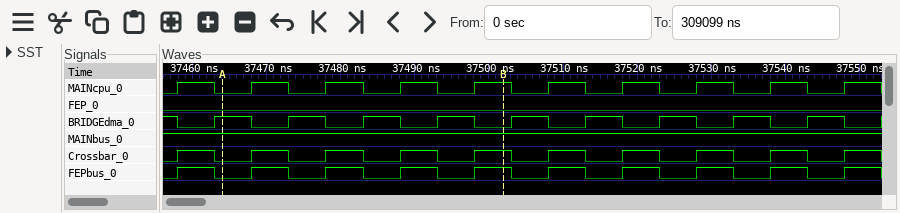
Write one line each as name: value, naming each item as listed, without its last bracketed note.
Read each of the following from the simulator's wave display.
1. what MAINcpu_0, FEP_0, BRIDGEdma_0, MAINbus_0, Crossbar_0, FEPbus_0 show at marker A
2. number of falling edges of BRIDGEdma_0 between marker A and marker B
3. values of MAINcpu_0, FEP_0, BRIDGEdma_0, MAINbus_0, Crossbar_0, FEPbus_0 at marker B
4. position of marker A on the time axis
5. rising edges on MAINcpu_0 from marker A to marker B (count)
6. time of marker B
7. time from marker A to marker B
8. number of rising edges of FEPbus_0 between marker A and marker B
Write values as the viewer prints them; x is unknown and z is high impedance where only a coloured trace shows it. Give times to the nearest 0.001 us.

what MAINcpu_0, FEP_0, BRIDGEdma_0, MAINbus_0, Crossbar_0, FEPbus_0 show at marker A: MAINcpu_0=0, FEP_0=0, BRIDGEdma_0=1, MAINbus_0=1, Crossbar_0=0, FEPbus_0=0
number of falling edges of BRIDGEdma_0 between marker A and marker B: 4
values of MAINcpu_0, FEP_0, BRIDGEdma_0, MAINbus_0, Crossbar_0, FEPbus_0 at marker B: MAINcpu_0=1, FEP_0=0, BRIDGEdma_0=0, MAINbus_0=1, Crossbar_0=1, FEPbus_0=1
position of marker A on the time axis: 37.464 us
rising edges on MAINcpu_0 from marker A to marker B: 4
time of marker B: 37.502 us
time from marker A to marker B: 0.038 us
number of rising edges of FEPbus_0 between marker A and marker B: 4
